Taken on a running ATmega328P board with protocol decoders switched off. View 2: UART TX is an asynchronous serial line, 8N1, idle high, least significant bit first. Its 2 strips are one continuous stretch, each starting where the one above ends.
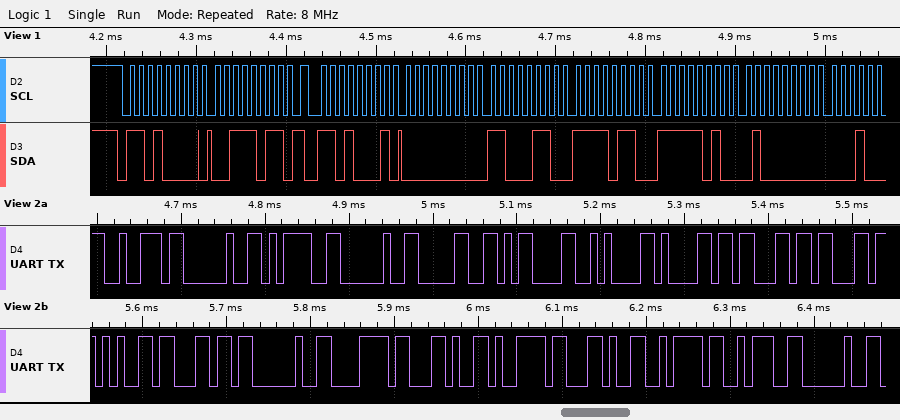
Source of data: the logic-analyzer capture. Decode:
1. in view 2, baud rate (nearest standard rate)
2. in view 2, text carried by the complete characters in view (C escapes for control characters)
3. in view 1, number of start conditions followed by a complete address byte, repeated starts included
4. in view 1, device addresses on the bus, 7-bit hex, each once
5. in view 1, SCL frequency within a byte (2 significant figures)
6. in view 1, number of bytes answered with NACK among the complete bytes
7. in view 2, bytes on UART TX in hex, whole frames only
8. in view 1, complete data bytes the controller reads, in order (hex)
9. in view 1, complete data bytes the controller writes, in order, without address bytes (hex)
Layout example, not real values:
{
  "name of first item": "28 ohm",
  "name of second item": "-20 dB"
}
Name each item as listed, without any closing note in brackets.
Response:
{
  "in view 2, baud rate": "115200 baud",
  "in view 2, text carried by the complete characters in view": "\"r = 0\\r\\naccel x,y,z: \"",
  "in view 1, number of start conditions followed by a complete address byte, repeated starts included": "2",
  "in view 1, device addresses on the bus, 7-bit hex, each once": "0x68",
  "in view 1, SCL frequency within a byte": "100 kHz",
  "in view 1, number of bytes answered with NACK among the complete bytes": "0",
  "in view 2, bytes on UART TX in hex, whole frames only": "0x72 0x20 0x3D 0x20 0x30 0x0D 0x0A 0x61 0x63 0x63 0x65 0x6C 0x20 0x78 0x2C 0x79 0x2C 0x7A 0x3A 0x20",
  "in view 1, complete data bytes the controller reads, in order": "00 C6 F6 FA 40",
  "in view 1, complete data bytes the controller writes, in order, without address bytes": "3B"
}
